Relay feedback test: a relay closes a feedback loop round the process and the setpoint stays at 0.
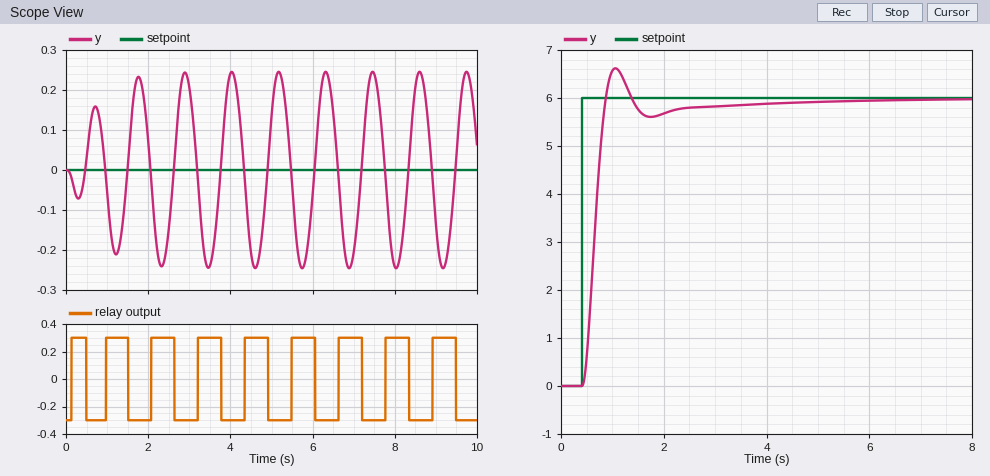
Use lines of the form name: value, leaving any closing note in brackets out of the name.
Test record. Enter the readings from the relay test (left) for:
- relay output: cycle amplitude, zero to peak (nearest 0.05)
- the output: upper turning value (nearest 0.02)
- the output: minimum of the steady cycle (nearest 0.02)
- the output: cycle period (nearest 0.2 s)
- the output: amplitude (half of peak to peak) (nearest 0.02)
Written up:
relay output: cycle amplitude, zero to peak: 0.30
the output: upper turning value: 0.24
the output: minimum of the steady cycle: -0.24
the output: cycle period: 1.2 s
the output: amplitude (half of peak to peak): 0.24
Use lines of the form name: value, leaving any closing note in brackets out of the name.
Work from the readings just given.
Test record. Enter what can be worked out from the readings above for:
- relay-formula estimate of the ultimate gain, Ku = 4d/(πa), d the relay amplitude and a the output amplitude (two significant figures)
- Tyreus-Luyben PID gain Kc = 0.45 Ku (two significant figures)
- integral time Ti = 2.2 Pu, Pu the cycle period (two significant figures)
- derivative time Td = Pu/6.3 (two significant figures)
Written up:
relay-formula estimate of the ultimate gain, Ku = 4d/(πa), d the relay amplitude and a the output amplitude: 1.6
Tyreus-Luyben PID gain Kc = 0.45 Ku: 0.72
integral time Ti = 2.2 Pu, Pu the cycle period: 2.6 s
derivative time Td = Pu/6.3: 0.19 s
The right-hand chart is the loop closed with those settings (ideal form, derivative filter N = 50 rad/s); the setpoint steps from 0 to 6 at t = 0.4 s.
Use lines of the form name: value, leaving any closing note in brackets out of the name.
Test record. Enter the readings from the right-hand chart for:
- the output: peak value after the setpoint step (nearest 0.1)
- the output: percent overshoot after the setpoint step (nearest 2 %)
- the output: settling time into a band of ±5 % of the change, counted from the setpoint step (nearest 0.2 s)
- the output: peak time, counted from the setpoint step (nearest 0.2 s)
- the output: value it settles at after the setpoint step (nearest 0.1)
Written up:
the output: peak value after the setpoint step: 6.6
the output: percent overshoot after the setpoint step: 10 %
the output: settling time into a band of ±5 % of the change, counted from the setpoint step: 1.6 s
the output: peak time, counted from the setpoint step: 0.6 s
the output: value it settles at after the setpoint step: 6.0
